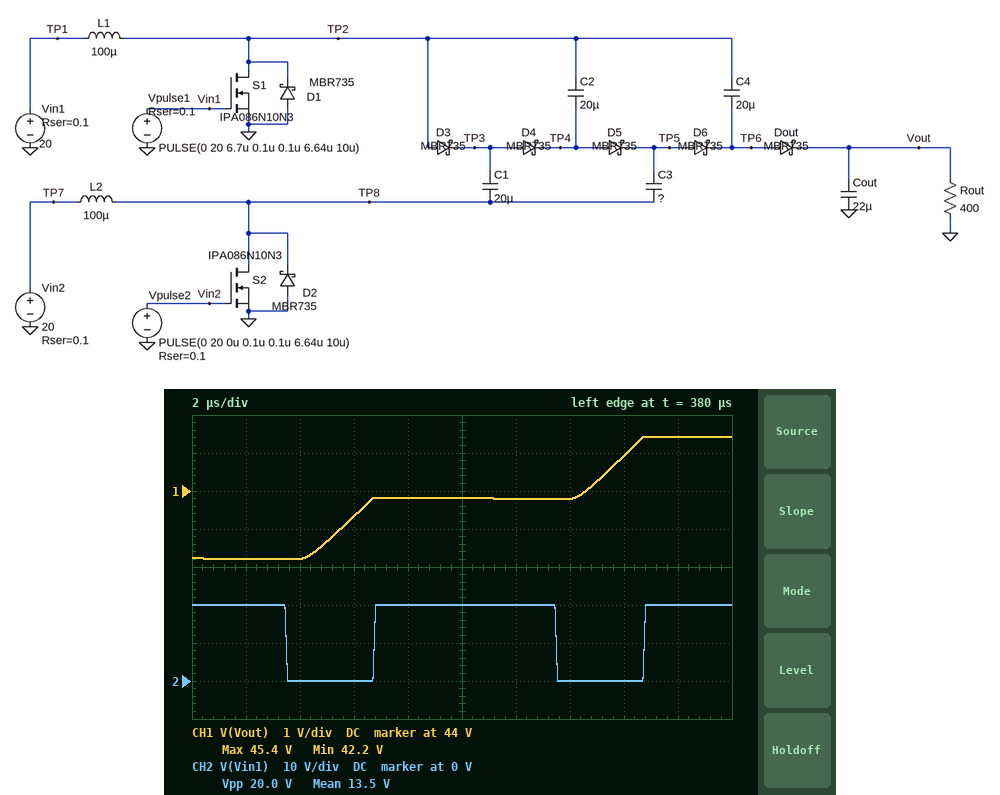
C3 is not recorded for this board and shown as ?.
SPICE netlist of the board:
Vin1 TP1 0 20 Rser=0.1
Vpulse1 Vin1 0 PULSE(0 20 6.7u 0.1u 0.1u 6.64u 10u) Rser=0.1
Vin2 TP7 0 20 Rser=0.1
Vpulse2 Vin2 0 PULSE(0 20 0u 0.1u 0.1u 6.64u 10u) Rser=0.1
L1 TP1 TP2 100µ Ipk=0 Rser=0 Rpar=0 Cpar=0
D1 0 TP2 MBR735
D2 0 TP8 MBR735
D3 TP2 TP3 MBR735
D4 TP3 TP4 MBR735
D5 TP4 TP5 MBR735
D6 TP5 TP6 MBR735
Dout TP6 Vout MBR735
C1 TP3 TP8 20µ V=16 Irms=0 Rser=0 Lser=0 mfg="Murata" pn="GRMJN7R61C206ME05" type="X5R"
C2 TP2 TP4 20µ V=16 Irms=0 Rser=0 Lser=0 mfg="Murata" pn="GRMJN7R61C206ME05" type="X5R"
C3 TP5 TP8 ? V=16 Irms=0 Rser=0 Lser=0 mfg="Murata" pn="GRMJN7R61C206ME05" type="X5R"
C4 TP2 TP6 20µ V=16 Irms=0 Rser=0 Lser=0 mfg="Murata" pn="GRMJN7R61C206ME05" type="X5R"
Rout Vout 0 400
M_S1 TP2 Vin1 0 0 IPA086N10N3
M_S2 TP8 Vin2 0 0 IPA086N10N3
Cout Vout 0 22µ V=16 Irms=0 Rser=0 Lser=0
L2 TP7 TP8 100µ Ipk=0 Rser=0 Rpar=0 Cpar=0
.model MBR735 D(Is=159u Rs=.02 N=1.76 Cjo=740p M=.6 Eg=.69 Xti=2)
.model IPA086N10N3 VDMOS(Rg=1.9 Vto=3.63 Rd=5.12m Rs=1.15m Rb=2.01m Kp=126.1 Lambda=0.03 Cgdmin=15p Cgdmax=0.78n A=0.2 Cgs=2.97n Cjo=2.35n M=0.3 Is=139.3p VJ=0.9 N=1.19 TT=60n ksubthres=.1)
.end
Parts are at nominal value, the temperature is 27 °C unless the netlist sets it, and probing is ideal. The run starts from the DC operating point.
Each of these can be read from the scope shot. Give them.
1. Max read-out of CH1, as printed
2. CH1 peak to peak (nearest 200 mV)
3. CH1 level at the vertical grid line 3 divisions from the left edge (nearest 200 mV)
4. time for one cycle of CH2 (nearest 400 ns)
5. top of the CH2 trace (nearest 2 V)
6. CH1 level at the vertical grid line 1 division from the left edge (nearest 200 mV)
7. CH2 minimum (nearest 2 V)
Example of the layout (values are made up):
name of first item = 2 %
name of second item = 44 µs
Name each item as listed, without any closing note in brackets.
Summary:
Max read-out of CH1, as printed = 45.4 V
CH1 peak to peak = 3.2 V
CH1 level at the vertical grid line 3 divisions from the left edge = 43.4 V
time for one cycle of CH2 = 10.0 µs
top of the CH2 trace = 20 V
CH1 level at the vertical grid line 1 division from the left edge = 42.2 V
CH2 minimum = 0 V
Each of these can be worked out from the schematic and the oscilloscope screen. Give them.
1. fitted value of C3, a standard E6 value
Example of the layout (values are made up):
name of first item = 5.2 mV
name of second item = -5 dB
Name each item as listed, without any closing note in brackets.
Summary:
fitted value of C3, a standard E6 value = 33 µF
